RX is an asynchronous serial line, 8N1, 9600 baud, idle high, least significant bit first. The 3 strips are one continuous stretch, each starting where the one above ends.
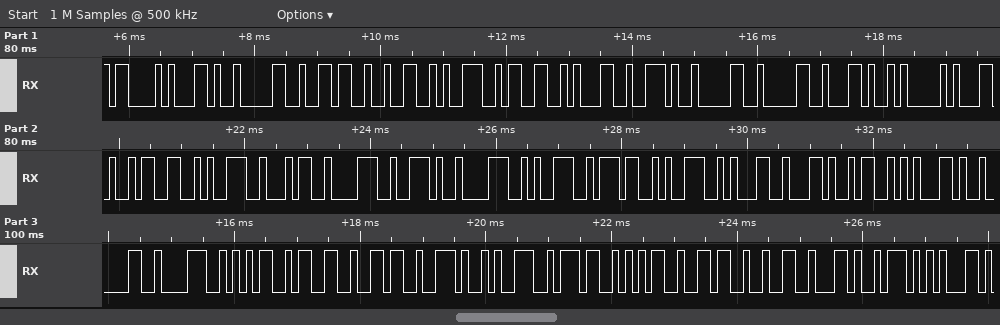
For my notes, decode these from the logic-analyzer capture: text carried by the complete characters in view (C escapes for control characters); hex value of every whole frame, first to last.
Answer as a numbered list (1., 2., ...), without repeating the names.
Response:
1. "C,062931.00,A,3948.89791,S,08536.97562,W"
2. 0x43 0x2C 0x30 0x36 0x32 0x39 0x33 0x31 0x2E 0x30 0x30 0x2C 0x41 0x2C 0x33 0x39 0x34 0x38 0x2E 0x38 0x39 0x37 0x39 0x31 0x2C 0x53 0x2C 0x30 0x38 0x35 0x33 0x36 0x2E 0x39 0x37 0x35 0x36 0x32 0x2C 0x57
